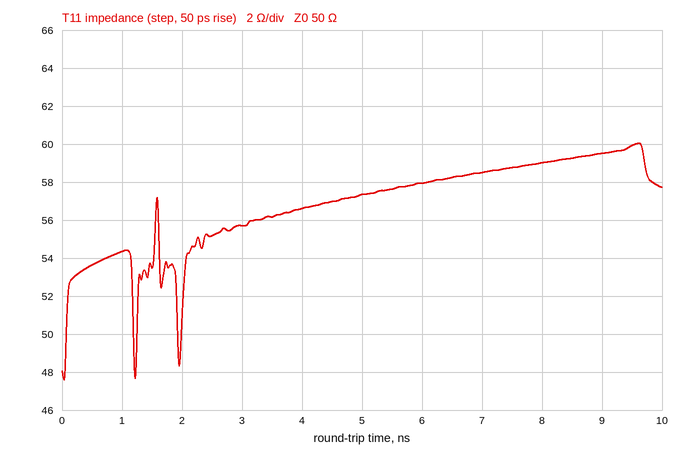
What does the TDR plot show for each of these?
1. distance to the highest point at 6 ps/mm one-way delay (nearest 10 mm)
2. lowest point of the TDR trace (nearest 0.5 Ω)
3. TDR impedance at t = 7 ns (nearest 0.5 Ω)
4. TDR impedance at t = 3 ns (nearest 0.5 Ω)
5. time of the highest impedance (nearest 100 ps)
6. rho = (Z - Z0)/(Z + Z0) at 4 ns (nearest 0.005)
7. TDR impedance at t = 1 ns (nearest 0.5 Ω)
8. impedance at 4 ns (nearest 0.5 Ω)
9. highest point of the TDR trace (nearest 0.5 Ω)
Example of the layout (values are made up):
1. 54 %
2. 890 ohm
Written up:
1. 800 mm
2. 47.5 Ω
3. 58.5 Ω
4. 55.5 Ω
5. 9.6 ns
6. +0.060
7. 54.5 Ω
8. 56.5 Ω
9. 60.0 Ω
